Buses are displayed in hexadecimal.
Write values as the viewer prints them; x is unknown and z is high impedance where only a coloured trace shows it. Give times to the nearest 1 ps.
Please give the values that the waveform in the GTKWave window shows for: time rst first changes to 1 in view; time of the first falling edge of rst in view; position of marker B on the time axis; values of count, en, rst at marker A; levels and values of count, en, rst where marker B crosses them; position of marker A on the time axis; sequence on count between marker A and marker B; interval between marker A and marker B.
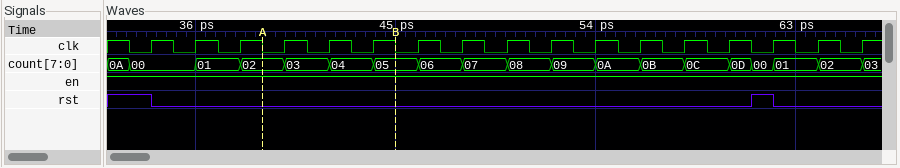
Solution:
61 ps
34 ps
45 ps
count=02, en=1, rst=0
count=05, en=1, rst=0
39 ps
02, 03, 04, 05
6 ps
